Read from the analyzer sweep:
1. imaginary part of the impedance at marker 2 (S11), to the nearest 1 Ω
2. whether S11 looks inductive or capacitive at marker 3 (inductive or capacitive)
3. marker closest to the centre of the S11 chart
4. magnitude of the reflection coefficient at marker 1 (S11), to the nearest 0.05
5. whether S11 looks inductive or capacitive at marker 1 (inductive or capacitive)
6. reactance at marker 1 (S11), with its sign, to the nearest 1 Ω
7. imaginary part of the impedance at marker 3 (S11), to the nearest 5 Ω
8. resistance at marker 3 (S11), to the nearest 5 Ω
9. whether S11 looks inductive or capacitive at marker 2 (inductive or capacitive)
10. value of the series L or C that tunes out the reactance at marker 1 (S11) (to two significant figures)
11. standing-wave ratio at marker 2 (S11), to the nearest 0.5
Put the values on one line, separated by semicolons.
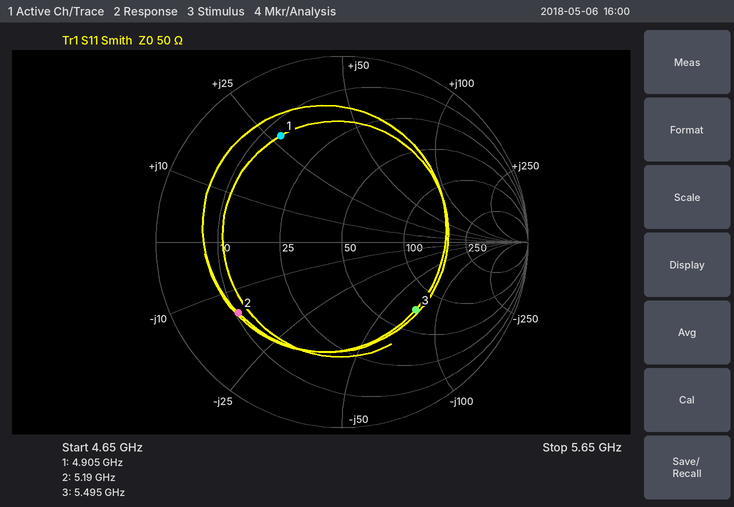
-15 Ω; capacitive; marker 3; 0.65; inductive; +27 Ω; -75 Ω; 70 Ω; capacitive; 1.2 pF; 5.0
